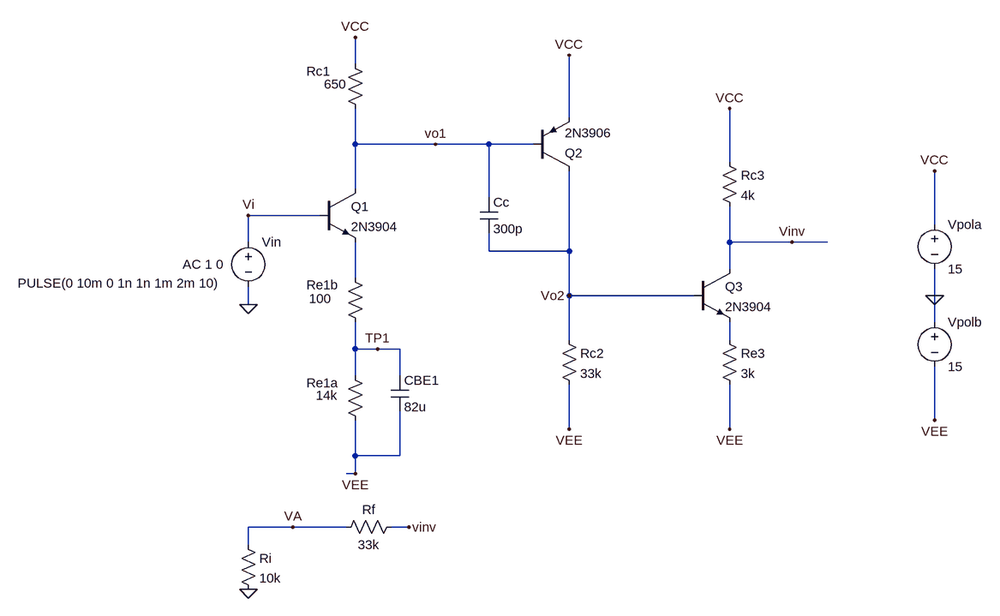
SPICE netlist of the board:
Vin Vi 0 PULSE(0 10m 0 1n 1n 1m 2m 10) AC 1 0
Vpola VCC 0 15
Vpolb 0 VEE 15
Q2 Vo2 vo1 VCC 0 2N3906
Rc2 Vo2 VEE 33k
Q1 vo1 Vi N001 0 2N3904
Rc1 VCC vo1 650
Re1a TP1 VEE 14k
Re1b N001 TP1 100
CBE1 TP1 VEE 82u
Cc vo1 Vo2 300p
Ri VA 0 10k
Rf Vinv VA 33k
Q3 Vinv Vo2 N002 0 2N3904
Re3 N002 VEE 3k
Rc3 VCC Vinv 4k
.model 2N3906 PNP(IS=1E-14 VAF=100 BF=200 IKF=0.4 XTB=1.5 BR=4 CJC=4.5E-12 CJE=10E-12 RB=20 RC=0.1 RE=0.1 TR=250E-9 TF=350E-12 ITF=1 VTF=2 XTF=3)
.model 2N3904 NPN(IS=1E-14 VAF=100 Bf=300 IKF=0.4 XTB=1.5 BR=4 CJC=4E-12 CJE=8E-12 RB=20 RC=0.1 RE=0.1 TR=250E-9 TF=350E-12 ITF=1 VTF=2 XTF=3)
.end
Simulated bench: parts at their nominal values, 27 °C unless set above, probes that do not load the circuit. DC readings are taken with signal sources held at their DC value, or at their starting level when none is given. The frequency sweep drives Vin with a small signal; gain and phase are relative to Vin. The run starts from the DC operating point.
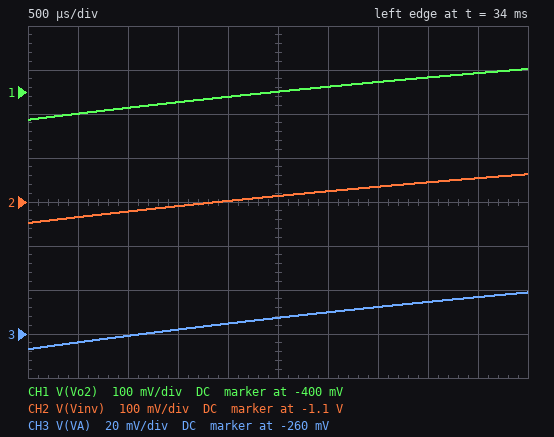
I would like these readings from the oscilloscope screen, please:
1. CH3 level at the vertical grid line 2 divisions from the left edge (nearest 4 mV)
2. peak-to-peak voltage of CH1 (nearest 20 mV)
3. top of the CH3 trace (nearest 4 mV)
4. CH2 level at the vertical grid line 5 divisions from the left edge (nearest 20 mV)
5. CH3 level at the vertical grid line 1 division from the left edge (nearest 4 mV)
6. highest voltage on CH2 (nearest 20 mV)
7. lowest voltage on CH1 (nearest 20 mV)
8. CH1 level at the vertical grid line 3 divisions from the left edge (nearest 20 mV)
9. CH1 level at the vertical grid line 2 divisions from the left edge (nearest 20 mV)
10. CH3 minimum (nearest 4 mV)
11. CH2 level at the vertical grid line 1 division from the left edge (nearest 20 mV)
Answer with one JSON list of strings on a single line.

["-260 mV", "120 mV", "-240 mV", "-1.08 V", "-264 mV", "-1.04 V", "-460 mV", "-420 mV", "-440 mV", "-268 mV", "-1.14 V"]
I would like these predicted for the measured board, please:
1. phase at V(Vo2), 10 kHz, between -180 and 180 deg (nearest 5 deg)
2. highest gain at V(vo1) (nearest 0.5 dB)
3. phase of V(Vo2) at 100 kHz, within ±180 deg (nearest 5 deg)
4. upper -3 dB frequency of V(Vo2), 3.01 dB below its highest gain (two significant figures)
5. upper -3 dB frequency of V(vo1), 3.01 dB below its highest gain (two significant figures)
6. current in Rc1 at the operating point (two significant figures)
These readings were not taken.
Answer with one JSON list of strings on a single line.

["-40 deg", "13.0 dB", "-85 deg", "12 kHz", "12 kHz", "1.0 mA"]
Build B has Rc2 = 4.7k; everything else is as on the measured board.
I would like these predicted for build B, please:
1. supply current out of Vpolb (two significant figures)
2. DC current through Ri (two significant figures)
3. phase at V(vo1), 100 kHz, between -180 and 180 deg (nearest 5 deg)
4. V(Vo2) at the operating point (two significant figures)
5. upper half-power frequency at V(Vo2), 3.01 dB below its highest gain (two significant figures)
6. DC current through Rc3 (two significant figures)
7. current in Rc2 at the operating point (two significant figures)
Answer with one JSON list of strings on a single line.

["4.0 mA", "170 µA", "135 deg", "-9.1 V", "4.1 kHz", "1.9 mA", "1.3 mA"]
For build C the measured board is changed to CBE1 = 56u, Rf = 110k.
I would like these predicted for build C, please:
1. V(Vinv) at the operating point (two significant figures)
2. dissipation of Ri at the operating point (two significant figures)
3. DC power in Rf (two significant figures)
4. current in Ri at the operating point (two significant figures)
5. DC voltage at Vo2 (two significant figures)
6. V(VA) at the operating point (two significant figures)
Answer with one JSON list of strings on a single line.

["-870 mV", "520 nW", "5.7 µW", "7.2 µA", "-170 mV", "-72 mV"]
